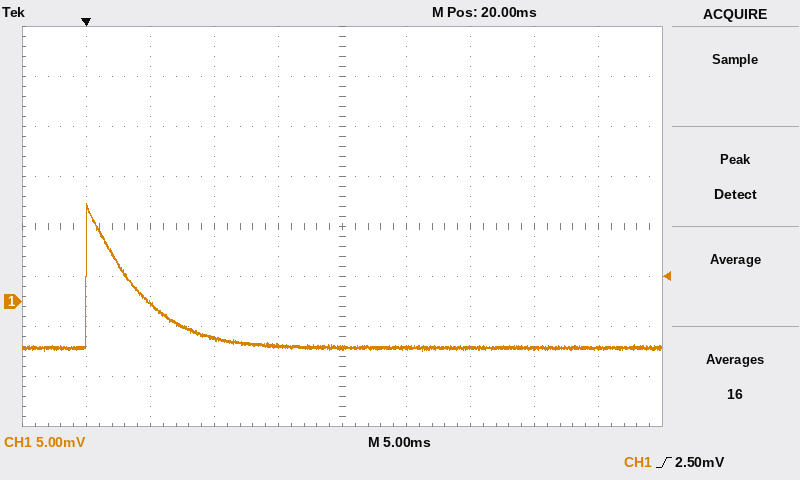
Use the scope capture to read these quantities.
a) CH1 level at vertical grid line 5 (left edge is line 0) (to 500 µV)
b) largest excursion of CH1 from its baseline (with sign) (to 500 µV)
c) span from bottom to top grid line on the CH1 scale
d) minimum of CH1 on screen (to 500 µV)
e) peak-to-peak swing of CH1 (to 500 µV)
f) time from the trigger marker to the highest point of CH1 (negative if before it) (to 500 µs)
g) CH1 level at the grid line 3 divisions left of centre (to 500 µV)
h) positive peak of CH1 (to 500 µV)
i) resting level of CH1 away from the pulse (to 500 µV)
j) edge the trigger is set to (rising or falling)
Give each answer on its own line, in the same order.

-4.5 mV
+14.5 mV
40 mV
-5.0 mV
15.0 mV
0.0 ms
0.0 mV
10.0 mV
-4.5 mV
rising
